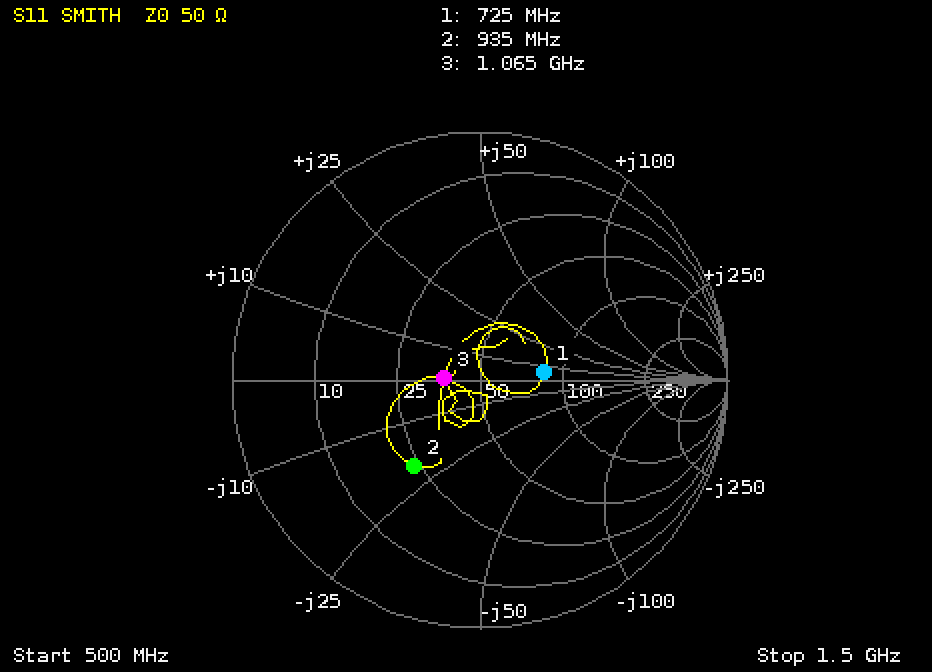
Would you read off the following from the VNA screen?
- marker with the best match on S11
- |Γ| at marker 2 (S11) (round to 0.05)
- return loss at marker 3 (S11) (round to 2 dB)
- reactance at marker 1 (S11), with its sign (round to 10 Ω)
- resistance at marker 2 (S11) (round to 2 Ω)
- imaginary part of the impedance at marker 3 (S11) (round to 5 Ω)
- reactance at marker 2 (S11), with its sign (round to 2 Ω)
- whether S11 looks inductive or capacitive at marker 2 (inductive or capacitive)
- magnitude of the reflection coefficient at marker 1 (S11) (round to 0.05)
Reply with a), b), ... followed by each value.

a) marker 3
b) 0.45
c) 16 dB
d) +10 Ω
e) 24 Ω
f) 0 Ω
g) -20 Ω
h) capacitive
i) 0.25
